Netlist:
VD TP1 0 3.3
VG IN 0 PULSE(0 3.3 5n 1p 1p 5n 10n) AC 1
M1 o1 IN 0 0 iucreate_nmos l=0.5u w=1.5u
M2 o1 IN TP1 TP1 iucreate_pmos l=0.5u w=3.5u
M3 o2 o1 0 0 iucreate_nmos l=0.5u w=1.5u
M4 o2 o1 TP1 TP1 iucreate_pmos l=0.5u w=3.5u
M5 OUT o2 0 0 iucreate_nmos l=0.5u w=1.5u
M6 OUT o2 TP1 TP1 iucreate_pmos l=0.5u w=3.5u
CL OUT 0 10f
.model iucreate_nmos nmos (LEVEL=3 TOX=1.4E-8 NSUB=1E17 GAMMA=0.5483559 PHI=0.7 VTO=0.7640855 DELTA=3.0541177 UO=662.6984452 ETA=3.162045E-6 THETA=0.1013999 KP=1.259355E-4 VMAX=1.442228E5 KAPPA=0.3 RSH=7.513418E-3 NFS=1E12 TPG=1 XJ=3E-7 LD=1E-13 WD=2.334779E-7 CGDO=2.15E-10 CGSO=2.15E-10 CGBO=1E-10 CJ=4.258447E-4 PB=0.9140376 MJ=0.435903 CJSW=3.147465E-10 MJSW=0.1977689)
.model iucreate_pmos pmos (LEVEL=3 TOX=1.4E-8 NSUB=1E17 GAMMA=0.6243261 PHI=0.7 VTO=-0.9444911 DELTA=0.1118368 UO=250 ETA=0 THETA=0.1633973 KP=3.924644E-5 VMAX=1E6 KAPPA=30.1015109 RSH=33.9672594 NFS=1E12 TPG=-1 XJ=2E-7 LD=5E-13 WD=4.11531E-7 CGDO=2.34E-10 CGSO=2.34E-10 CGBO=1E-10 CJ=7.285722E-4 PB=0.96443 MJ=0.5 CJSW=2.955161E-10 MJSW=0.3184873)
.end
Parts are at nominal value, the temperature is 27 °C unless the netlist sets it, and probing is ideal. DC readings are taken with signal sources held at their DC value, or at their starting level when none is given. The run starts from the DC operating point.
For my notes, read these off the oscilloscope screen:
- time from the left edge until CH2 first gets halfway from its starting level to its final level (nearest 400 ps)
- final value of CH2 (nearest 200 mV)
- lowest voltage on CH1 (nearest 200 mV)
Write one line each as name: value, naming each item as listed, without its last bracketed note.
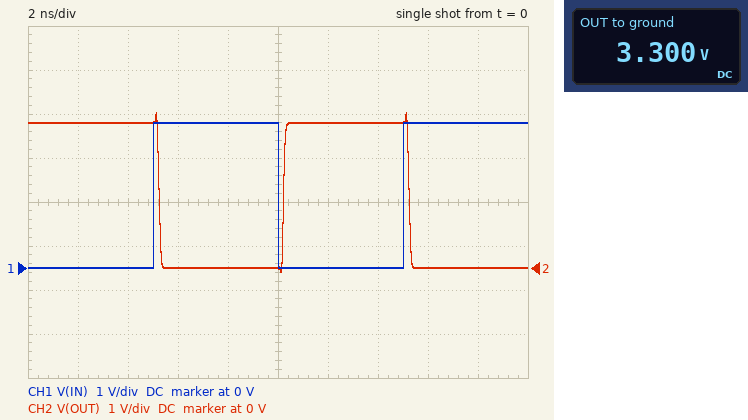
time from the left edge until CH2 first gets halfway from its starting level to its final level: 5.2 ns
final value of CH2: 0 V
lowest voltage on CH1: 0 V
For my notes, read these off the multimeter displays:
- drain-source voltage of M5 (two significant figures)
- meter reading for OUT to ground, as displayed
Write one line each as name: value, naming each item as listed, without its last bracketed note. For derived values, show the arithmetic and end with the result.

drain-source voltage of M5: 3.3 V = 3.3 V
meter reading for OUT to ground, as displayed: 3.300 V
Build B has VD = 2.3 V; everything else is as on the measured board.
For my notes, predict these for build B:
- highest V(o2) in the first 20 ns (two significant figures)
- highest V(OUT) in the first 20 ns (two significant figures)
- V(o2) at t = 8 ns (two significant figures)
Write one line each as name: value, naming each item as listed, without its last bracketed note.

highest V(o2) in the first 20 ns: 2.6 V
highest V(OUT) in the first 20 ns: 2.5 V
V(o2) at t = 8 ns: 2.3 V
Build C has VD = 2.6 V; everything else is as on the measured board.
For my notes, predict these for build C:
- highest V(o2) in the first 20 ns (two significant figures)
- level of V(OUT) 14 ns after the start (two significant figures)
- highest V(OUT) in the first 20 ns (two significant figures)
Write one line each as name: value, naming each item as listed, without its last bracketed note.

highest V(o2) in the first 20 ns: 2.9 V
level of V(OUT) 14 ns after the start: 2.6 V
highest V(OUT) in the first 20 ns: 2.8 V
